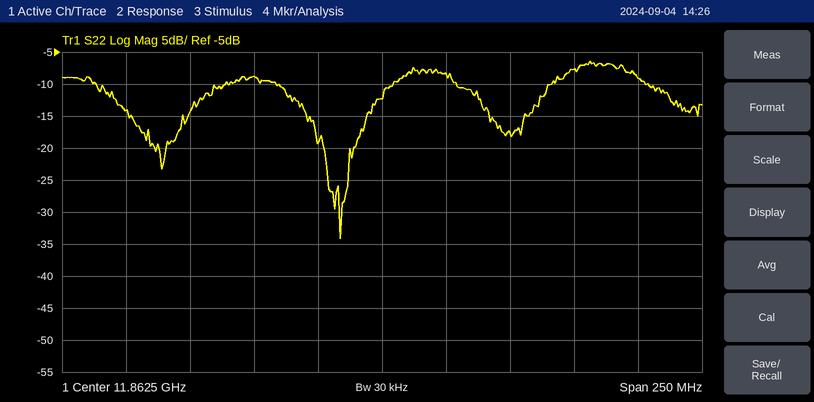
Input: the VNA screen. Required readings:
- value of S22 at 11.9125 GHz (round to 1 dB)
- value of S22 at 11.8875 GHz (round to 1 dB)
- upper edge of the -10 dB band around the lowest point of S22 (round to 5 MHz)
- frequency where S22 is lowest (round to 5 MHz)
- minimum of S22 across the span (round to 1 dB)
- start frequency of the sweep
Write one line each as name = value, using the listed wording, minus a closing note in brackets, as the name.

value of S22 at 11.9125 GHz = -18 dB
value of S22 at 11.8875 GHz = -8 dB
upper edge of the -10 dB band around the lowest point of S22 = 11.865 GHz
frequency where S22 is lowest = 11.845 GHz
minimum of S22 across the span = -34 dB
start frequency of the sweep = 11.7375 GHz
